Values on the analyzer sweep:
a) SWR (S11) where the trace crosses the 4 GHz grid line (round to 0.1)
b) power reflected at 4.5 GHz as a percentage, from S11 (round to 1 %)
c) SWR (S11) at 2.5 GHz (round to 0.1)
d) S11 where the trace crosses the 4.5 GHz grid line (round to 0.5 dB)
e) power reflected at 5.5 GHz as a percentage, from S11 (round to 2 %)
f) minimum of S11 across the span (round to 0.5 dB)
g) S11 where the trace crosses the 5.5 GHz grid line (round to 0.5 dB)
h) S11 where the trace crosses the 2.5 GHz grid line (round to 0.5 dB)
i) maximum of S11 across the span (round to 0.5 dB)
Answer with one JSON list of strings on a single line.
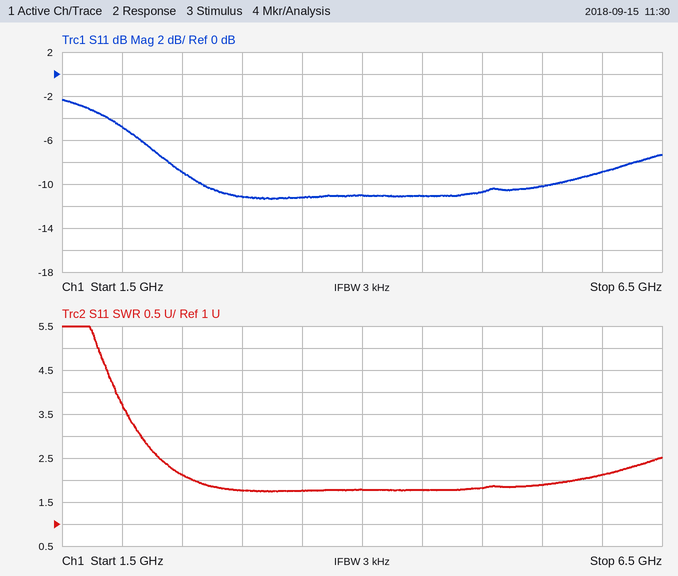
["1.8", "8 %", "2.1", "-11.0 dB", "10 %", "-11.5 dB", "-10.0 dB", "-9.0 dB", "-2.5 dB"]
